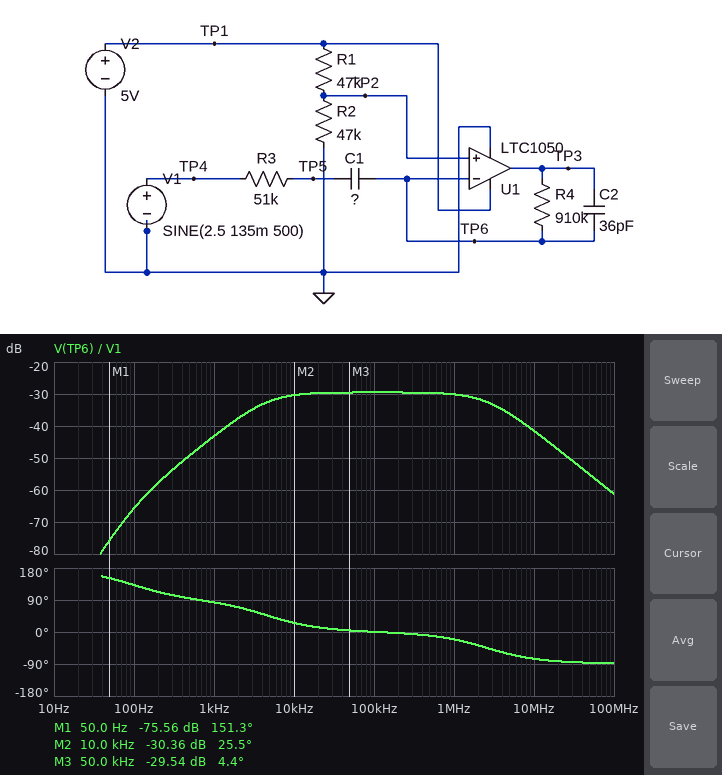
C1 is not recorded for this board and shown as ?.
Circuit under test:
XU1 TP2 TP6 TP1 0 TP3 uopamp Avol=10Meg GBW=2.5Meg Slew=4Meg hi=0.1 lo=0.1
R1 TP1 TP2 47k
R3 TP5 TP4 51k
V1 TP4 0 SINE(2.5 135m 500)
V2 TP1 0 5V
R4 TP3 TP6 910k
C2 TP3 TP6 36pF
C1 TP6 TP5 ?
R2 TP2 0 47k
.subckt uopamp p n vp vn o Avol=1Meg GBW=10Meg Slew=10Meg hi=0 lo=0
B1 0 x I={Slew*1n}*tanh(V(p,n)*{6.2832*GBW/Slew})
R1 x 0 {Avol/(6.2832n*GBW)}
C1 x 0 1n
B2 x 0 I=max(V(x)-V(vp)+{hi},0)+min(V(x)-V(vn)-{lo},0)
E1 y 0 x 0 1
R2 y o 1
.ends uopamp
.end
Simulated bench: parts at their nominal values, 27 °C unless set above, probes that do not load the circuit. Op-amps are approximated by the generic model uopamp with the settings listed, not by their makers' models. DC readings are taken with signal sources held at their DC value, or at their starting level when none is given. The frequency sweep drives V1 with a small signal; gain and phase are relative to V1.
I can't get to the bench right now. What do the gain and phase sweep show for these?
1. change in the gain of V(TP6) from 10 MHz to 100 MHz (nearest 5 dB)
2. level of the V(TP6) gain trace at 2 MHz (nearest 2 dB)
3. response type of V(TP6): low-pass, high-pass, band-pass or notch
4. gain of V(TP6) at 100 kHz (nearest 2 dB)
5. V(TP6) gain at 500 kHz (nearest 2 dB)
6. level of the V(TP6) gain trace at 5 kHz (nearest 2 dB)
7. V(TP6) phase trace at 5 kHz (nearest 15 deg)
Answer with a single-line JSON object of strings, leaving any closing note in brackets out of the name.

{"change in the gain of V(TP6) from 10 MHz to 100 MHz": "-20 dB", "level of the V(TP6) gain trace at 2 MHz": "-32 dB", "response type of V(TP6): low-pass, high-pass, band-pass or notch": "band-pass", "gain of V(TP6) at 100 kHz": "-30 dB", "V(TP6) gain at 500 kHz": "-30 dB", "level of the V(TP6) gain trace at 5 kHz": "-32 dB", "V(TP6) phase trace at 5 kHz": "45 deg"}
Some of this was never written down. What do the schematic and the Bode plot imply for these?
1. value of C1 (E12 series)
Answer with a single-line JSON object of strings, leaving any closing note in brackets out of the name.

{"value of C1": "33 nF"}
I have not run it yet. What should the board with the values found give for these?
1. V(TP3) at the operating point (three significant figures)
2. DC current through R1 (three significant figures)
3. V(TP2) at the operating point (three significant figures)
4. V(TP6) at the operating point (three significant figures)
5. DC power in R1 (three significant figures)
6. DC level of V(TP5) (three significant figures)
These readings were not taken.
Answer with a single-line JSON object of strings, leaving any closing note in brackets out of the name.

{"V(TP3) at the operating point": "2.50 V", "DC current through R1": "53.2 µA", "V(TP2) at the operating point": "2.50 V", "V(TP6) at the operating point": "2.50 V", "DC power in R1": "133 µW", "DC level of V(TP5)": "2.50 V"}
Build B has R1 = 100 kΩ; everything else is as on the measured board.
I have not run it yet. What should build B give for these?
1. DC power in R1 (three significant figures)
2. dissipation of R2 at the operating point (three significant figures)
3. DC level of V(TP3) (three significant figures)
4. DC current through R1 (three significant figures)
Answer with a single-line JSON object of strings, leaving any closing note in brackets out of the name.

{"DC power in R1": "116 µW", "dissipation of R2 at the operating point": "54.4 µW", "DC level of V(TP3)": "1.60 V", "DC current through R1": "34.0 µA"}
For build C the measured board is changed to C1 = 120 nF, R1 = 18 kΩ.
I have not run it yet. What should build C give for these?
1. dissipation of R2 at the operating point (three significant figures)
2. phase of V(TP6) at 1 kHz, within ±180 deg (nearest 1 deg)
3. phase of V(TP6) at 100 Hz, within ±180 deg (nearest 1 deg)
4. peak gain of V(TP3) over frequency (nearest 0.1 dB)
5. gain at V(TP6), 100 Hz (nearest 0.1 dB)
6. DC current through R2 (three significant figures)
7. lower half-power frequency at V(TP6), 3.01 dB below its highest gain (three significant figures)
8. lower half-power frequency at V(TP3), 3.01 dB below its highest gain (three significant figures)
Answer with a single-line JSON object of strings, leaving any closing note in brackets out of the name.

{"dissipation of R2 at the operating point": "278 µW", "phase of V(TP6) at 1 kHz, within ±180 deg": "79 deg", "phase of V(TP6) at 100 Hz, within ±180 deg": "103 deg", "peak gain of V(TP3) over frequency": "25.0 dB", "gain at V(TP6), 100 Hz": "-63.2 dB", "DC current through R2": "76.9 µA", "lower half-power frequency at V(TP6), 3.01 dB below its highest gain": "4.68 kHz", "lower half-power frequency at V(TP3), 3.01 dB below its highest gain": "25.7 Hz"}
